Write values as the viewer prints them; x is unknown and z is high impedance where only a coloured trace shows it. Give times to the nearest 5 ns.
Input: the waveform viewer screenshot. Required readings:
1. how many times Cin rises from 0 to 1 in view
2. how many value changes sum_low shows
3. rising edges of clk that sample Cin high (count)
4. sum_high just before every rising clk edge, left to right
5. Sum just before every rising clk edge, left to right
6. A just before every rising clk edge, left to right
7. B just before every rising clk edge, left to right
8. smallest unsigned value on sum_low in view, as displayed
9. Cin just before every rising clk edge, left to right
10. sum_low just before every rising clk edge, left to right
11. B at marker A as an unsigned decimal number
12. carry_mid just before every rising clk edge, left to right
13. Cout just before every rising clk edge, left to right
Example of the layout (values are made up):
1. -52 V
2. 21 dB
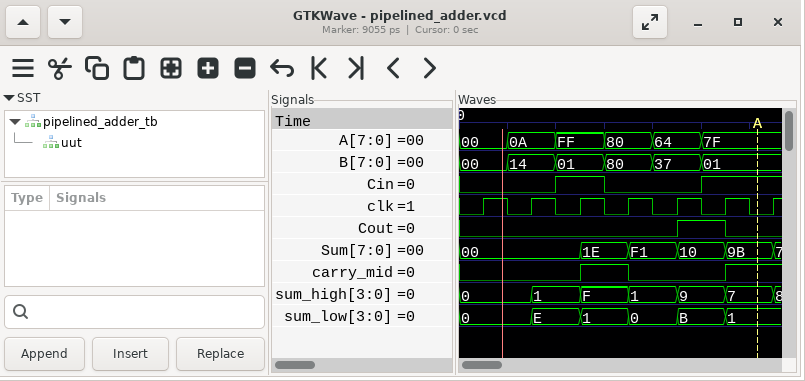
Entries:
1. 2
2. 5
3. 3
4. 0, 0, 1, F, 1, 9, 7
5. 00, 00, 00, 1E, F1, 10, 9B
6. 00, 0A, FF, 80, 64, 7F, 7F
7. 00, 14, 01, 80, 37, 01, 01
8. 0
9. 0 0 1 0 0 1 1
10. 0, 0, E, 1, 0, B, 1
11. 1
12. 0 0 0 1 0 0 1
13. 0 0 0 0 0 1 0
